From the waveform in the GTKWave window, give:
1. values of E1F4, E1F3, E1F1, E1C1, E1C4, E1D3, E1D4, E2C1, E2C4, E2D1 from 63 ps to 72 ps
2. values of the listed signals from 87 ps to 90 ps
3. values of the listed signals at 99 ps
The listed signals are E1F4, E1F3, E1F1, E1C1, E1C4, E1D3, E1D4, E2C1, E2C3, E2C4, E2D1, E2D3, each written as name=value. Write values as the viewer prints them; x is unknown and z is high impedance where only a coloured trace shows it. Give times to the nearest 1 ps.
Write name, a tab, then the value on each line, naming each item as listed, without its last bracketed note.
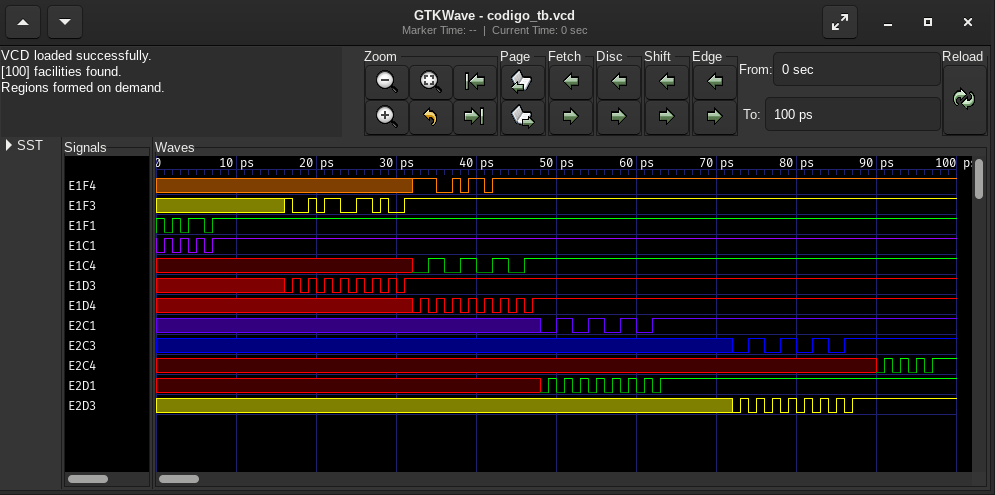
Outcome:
values of E1F4, E1F3, E1F1, E1C1, E1C4, E1D3, E1D4, E2C1, E2C4, E2D1 from 63 ps to 72 ps	E1F4=1, E1F3=1, E1F1=1, E1C1=1, E1C4=1, E1D3=1, E1D4=1, E2C1=1, E2C4=x, E2D1=1
values of the listed signals from 87 ps to 90 ps	E1F4=1, E1F3=1, E1F1=1, E1C1=1, E1C4=1, E1D3=1, E1D4=1, E2C1=1, E2C3=1, E2C4=x, E2D1=1, E2D3=1
values of the listed signals at 99 ps	E1F4=1, E1F3=1, E1F1=1, E1C1=1, E1C4=1, E1D3=1, E1D4=1, E2C1=1, E2C3=1, E2C4=1, E2D1=1, E2D3=1
